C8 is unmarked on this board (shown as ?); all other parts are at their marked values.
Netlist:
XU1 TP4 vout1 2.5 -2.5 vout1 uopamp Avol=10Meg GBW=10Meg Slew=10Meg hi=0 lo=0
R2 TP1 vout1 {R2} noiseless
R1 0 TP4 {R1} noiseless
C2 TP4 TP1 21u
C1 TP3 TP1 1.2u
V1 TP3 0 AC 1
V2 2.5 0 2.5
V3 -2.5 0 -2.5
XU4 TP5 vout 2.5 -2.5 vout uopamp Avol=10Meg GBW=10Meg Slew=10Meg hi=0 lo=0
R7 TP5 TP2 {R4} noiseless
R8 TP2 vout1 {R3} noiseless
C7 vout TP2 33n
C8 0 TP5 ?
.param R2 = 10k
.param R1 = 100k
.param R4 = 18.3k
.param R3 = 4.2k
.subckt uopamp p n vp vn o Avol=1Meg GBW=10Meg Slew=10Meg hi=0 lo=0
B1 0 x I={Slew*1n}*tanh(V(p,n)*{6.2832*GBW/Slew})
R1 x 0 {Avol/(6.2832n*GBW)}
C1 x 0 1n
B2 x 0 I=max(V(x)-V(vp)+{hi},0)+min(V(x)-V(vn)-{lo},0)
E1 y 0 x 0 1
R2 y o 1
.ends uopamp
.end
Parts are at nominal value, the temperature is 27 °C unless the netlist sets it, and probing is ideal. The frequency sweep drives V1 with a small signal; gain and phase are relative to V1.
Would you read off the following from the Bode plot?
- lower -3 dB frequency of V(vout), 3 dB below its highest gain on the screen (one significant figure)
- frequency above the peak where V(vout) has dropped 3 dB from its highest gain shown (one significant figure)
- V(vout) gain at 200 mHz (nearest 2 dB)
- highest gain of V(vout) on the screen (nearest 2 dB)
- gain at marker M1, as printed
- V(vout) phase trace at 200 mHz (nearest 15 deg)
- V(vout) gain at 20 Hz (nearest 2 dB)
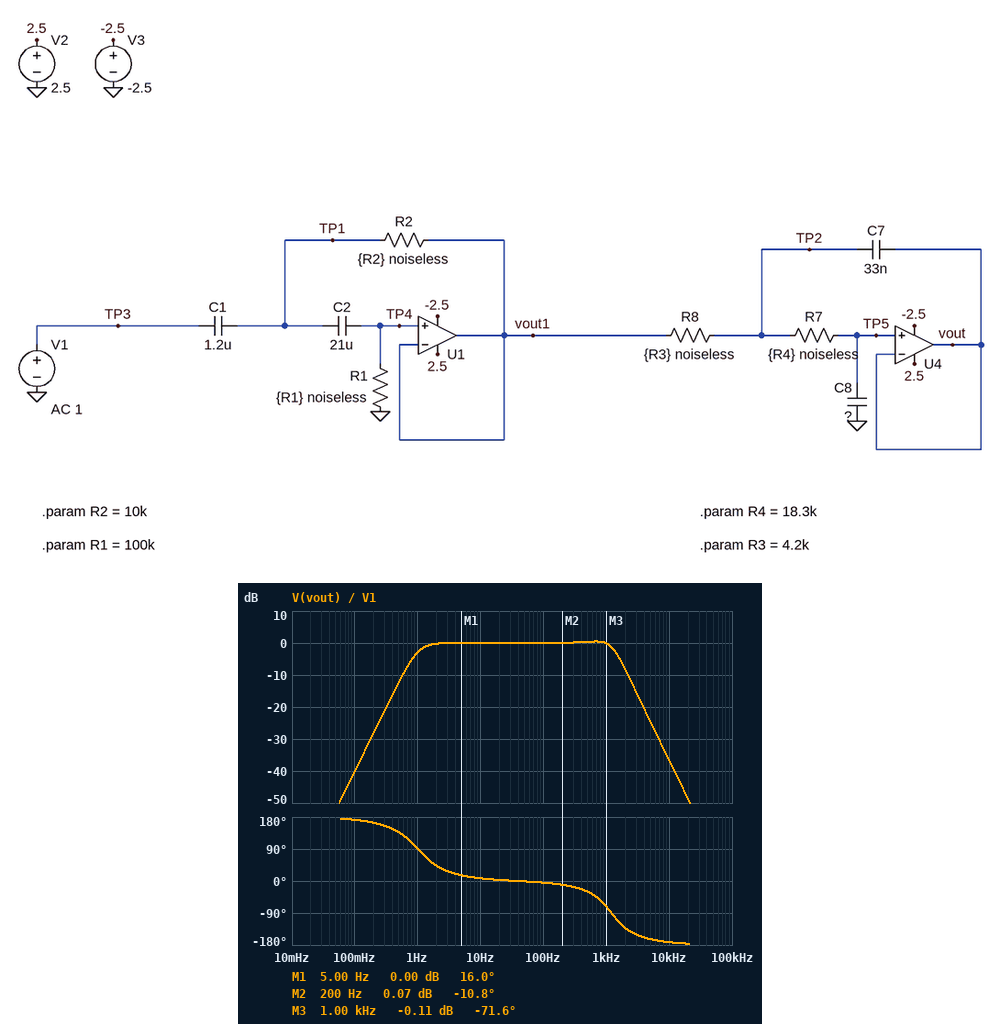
1 Hz
1 kHz
-28 dB
0 dB
0.00 dB
165 deg
0 dB
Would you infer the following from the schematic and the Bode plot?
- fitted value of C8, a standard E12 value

6.8 nF
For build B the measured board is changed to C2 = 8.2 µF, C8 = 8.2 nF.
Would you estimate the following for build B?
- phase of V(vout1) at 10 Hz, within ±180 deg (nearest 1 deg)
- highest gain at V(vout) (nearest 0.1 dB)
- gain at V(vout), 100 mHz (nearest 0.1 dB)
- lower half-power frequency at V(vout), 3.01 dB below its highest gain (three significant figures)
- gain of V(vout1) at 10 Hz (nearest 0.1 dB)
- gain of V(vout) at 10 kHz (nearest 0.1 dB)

9 deg
1.6 dB
-48.2 dB
1.36 Hz
0.1 dB
-38.3 dB
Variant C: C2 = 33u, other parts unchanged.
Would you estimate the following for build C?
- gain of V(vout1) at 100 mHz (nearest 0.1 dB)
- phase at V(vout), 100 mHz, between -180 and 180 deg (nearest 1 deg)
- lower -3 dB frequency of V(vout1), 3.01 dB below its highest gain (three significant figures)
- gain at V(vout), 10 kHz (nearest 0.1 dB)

-36.2 dB
168 deg
1.01 Hz
-36.6 dB
